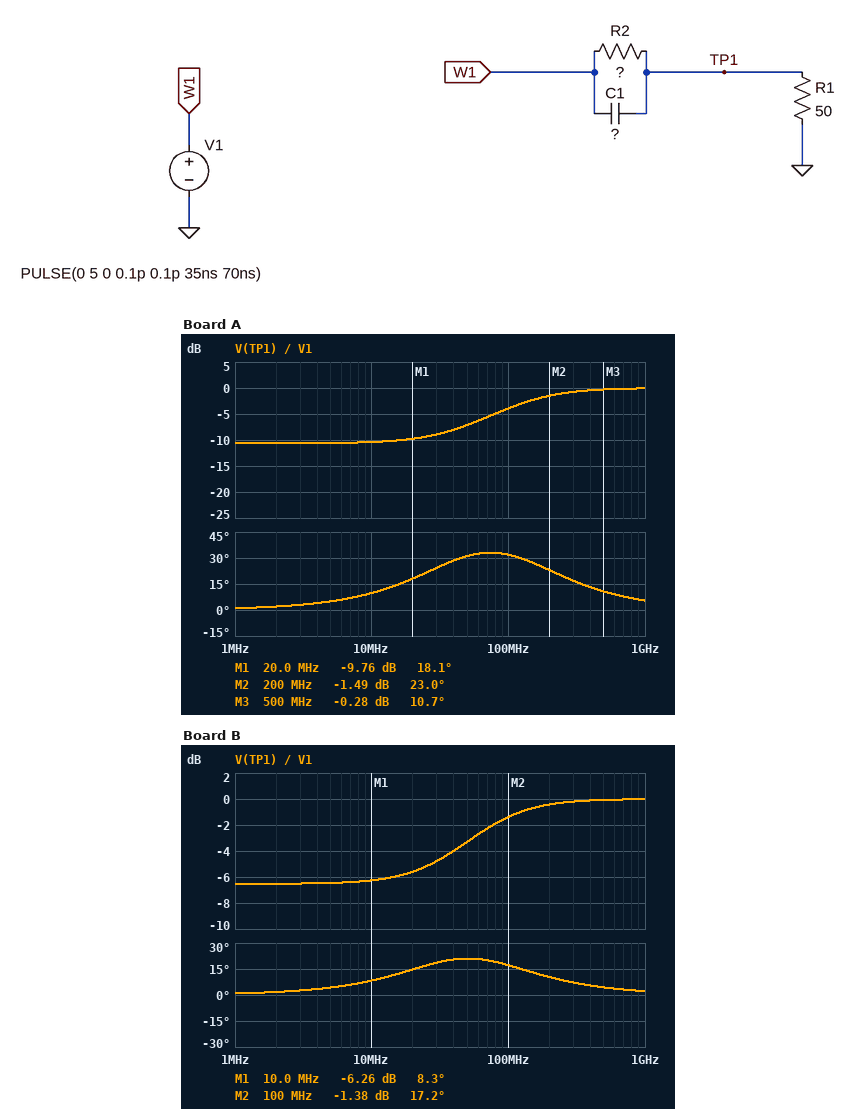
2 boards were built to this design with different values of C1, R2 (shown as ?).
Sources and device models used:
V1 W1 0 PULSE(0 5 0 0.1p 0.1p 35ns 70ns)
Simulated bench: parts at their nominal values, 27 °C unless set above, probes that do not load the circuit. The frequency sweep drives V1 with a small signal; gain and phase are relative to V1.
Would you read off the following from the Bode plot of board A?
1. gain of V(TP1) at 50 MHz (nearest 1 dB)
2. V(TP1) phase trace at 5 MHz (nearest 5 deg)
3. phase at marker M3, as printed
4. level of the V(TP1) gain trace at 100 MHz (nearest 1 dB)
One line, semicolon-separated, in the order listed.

-7 dB; 5 deg; 10.7 deg; -4 dB
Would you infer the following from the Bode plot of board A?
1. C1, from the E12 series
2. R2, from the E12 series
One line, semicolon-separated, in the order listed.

33 pF; 120 Ω
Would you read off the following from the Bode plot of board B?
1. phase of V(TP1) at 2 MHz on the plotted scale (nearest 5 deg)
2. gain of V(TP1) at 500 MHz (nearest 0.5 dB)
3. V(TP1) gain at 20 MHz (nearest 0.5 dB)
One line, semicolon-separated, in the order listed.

0 deg; 0 dB; -5.5 dB
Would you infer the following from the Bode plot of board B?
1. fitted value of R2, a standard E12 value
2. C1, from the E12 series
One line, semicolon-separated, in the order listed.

56 Ω; 82 pF
